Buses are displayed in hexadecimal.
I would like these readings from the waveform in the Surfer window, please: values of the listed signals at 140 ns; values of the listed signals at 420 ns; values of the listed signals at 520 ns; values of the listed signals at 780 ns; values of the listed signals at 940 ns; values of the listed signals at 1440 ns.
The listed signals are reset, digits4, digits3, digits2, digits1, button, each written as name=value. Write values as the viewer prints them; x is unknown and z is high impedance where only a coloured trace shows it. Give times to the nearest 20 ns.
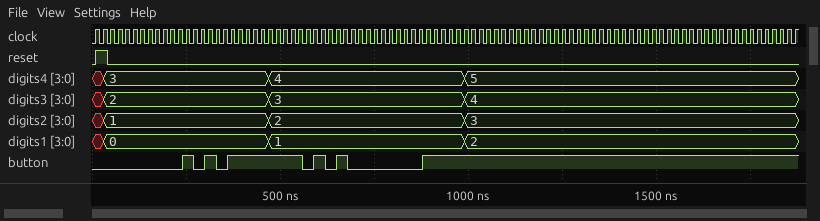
reset=0, digits4=3, digits3=2, digits2=1, digits1=0, button=0
reset=0, digits4=3, digits3=2, digits2=1, digits1=0, button=1
reset=0, digits4=4, digits3=3, digits2=2, digits1=1, button=1
reset=0, digits4=4, digits3=3, digits2=2, digits1=1, button=0
reset=0, digits4=4, digits3=3, digits2=2, digits1=1, button=1
reset=0, digits4=5, digits3=4, digits2=3, digits1=2, button=1
